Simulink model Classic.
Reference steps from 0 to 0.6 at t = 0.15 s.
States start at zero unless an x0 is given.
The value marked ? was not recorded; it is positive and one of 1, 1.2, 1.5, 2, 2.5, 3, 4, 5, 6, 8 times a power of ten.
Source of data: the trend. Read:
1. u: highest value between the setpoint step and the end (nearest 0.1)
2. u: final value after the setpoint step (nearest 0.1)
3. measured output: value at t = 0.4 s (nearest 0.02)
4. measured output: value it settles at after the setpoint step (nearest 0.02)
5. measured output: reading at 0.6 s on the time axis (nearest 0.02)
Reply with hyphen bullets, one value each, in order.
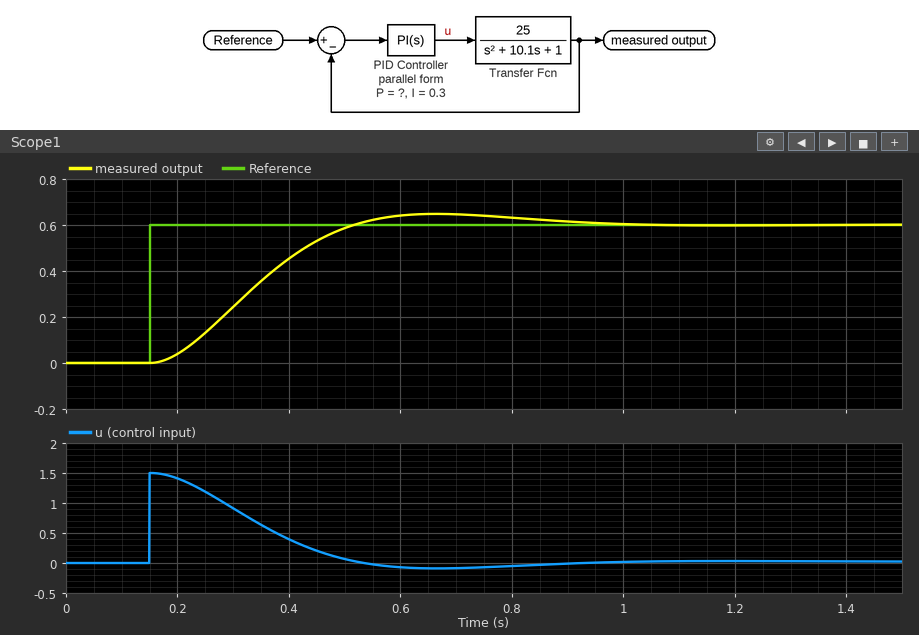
- 1.5
- 0.0
- 0.46
- 0.60
- 0.64
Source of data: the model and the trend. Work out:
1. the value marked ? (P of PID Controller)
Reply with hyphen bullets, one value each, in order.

- 2.5
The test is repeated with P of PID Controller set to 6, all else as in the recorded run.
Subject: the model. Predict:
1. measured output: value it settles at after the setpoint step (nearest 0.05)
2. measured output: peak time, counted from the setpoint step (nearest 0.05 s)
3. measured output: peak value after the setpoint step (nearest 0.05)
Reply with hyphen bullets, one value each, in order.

- 0.60
- 0.30 s
- 0.75
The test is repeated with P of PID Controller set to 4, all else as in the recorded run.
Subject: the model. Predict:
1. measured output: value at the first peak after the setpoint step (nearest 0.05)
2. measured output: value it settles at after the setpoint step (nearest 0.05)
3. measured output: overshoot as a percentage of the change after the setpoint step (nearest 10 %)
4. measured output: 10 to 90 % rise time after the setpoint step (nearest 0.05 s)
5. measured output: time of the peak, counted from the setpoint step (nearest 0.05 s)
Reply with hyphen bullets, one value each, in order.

- 0.70
- 0.60
- 20 %
- 0.15 s
- 0.35 s
